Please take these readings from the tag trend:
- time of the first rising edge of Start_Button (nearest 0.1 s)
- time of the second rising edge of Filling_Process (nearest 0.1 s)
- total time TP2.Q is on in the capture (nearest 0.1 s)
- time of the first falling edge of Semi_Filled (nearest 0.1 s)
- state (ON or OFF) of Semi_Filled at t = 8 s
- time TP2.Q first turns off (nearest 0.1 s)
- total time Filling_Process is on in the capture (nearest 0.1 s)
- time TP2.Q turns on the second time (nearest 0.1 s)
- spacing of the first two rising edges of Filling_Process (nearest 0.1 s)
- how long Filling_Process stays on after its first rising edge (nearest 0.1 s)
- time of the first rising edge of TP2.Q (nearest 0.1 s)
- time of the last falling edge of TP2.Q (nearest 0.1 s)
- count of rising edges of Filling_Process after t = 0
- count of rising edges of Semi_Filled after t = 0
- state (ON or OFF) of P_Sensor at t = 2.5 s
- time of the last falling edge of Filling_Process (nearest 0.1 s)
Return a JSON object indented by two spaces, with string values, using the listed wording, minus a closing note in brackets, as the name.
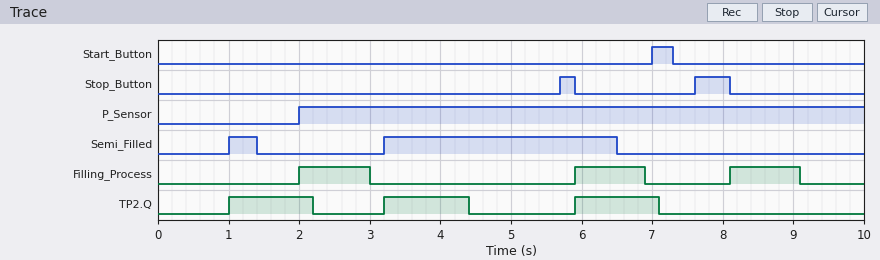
{
  "time of the first rising edge of Start_Button": "7.0 s",
  "time of the second rising edge of Filling_Process": "5.9 s",
  "total time TP2.Q is on in the capture": "3.6 s",
  "time of the first falling edge of Semi_Filled": "1.4 s",
  "state (ON or OFF) of Semi_Filled at t = 8 s": "OFF",
  "time TP2.Q first turns off": "2.2 s",
  "total time Filling_Process is on in the capture": "3.0 s",
  "time TP2.Q turns on the second time": "3.2 s",
  "spacing of the first two rising edges of Filling_Process": "3.9 s",
  "how long Filling_Process stays on after its first rising edge": "1.0 s",
  "time of the first rising edge of TP2.Q": "1.0 s",
  "time of the last falling edge of TP2.Q": "7.1 s",
  "count of rising edges of Filling_Process after t = 0": "3",
  "count of rising edges of Semi_Filled after t = 0": "2",
  "state (ON or OFF) of P_Sensor at t = 2.5 s": "ON",
  "time of the last falling edge of Filling_Process": "9.1 s"
}
